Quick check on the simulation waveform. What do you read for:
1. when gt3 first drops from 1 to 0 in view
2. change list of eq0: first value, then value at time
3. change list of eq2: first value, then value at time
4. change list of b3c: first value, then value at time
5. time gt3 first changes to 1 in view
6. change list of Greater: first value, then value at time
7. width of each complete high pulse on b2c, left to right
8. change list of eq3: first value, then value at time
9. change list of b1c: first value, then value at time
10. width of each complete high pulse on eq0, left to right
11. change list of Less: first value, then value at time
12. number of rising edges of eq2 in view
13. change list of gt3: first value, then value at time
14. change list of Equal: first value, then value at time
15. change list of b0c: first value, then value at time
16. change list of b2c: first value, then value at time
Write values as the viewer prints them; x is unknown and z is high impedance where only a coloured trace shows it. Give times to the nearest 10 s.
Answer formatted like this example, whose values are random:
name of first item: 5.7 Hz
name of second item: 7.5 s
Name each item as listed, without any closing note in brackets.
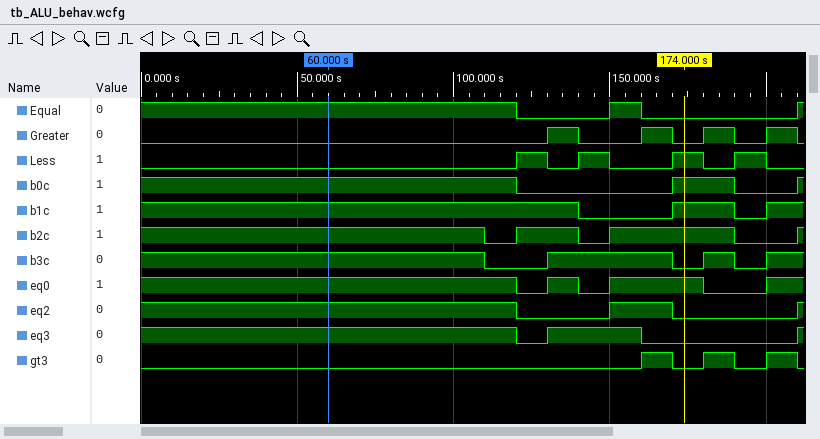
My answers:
when gt3 first drops from 1 to 0 in view: 170 s
change list of eq0: first value, then value at time: 1, 0 at 120 s, 1 at 130 s, 0 at 140 s, 1 at 150 s, 0 at 180 s, 1 at 200 s
change list of eq2: first value, then value at time: 1, 0 at 120 s, 1 at 150 s, 0 at 170 s, 1 at 210 s
change list of b3c: first value, then value at time: 1, 0 at 110 s, 1 at 130 s, 0 at 170 s, 1 at 180 s, 0 at 190 s, 1 at 200 s
time gt3 first changes to 1 in view: 160 s
change list of Greater: first value, then value at time: 0, 1 at 130 s, 0 at 140 s, 1 at 160 s, 0 at 170 s, 1 at 180 s, 0 at 190 s, 1 at 200 s, 0 at 210 s
width of each complete high pulse on b2c, left to right: 20 s, 40 s
change list of eq3: first value, then value at time: 1, 0 at 120 s, 1 at 130 s, 0 at 160 s, 1 at 210 s
change list of b1c: first value, then value at time: 1, 0 at 140 s, 1 at 170 s, 0 at 190 s, 1 at 200 s
width of each complete high pulse on eq0, left to right: 10 s, 30 s
change list of Less: first value, then value at time: 0, 1 at 120 s, 0 at 130 s, 1 at 140 s, 0 at 150 s, 1 at 170 s, 0 at 180 s, 1 at 190 s, 0 at 200 s
number of rising edges of eq2 in view: 2
change list of gt3: first value, then value at time: 0, 1 at 160 s, 0 at 170 s, 1 at 180 s, 0 at 190 s, 1 at 200 s, 0 at 210 s
change list of Equal: first value, then value at time: 1, 0 at 120 s, 1 at 150 s, 0 at 160 s, 1 at 210 s
change list of b0c: first value, then value at time: 1, 0 at 120 s, 1 at 170 s, 0 at 190 s, 1 at 210 s
change list of b2c: first value, then value at time: 1, 0 at 110 s, 1 at 120 s, 0 at 140 s, 1 at 150 s, 0 at 190 s, 1 at 210 s
